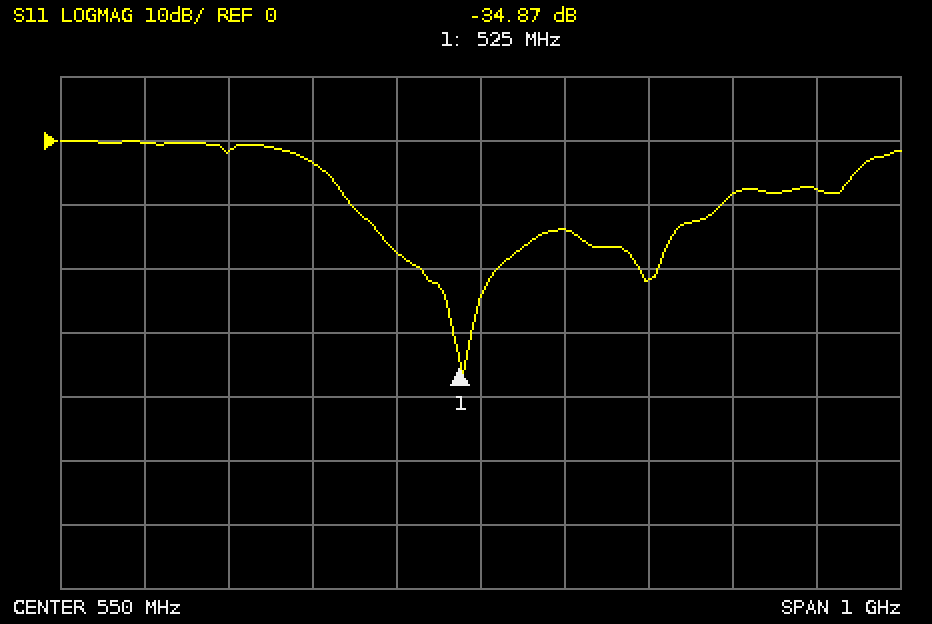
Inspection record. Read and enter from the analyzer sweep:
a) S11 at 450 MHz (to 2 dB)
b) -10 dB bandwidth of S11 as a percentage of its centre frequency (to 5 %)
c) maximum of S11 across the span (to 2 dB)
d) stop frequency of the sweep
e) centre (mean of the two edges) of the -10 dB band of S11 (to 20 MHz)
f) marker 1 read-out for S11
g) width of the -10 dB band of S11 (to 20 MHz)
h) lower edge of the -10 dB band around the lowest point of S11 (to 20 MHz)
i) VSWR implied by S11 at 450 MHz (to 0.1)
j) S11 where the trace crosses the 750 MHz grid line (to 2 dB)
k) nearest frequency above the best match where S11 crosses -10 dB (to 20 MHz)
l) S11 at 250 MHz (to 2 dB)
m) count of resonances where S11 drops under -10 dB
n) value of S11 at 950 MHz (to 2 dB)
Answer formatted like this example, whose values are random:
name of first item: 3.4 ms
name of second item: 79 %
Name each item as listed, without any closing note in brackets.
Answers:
S11 at 450 MHz: -18 dB
-10 dB bandwidth of S11 as a percentage of its centre frequency: 70 %
maximum of S11 across the span: 0 dB
stop frequency of the sweep: 1.05 GHz
centre (mean of the two edges) of the -10 dB band of S11: 620 MHz
marker 1 read-out for S11: -34.87 dB
width of the -10 dB band of S11: 440 MHz
lower edge of the -10 dB band around the lowest point of S11: 400 MHz
VSWR implied by S11 at 450 MHz: 1.3
S11 where the trace crosses the 750 MHz grid line: -22 dB
nearest frequency above the best match where S11 crosses -10 dB: 840 MHz
S11 at 250 MHz: -2 dB
count of resonances where S11 drops under -10 dB: 2
value of S11 at 950 MHz: -8 dB
